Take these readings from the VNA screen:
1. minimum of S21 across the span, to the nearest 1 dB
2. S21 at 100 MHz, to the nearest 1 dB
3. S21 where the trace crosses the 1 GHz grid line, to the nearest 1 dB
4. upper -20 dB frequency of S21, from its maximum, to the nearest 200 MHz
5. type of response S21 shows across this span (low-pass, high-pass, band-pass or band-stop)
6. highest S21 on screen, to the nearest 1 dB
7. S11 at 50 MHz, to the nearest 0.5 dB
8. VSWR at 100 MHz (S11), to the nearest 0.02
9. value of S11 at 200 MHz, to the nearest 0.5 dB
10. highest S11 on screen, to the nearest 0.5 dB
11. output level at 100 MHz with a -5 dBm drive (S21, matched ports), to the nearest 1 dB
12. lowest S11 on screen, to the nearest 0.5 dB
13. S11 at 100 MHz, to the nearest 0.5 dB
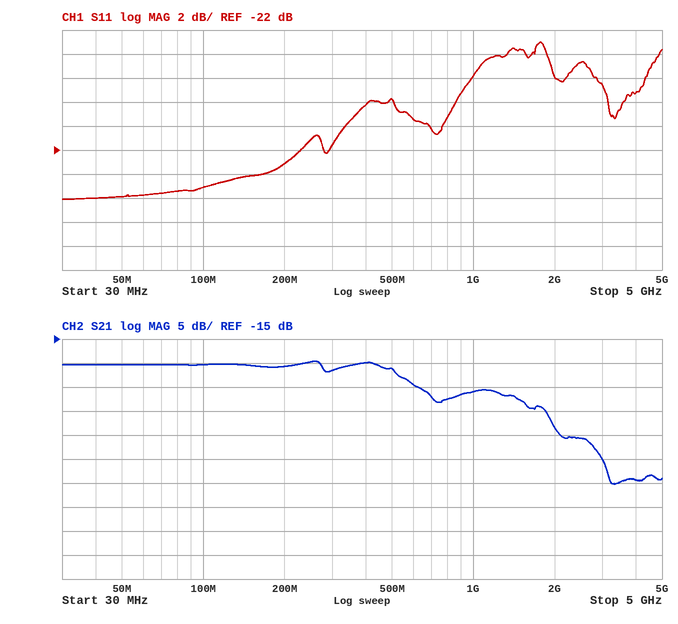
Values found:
-45 dB
-20 dB
-26 dB
3.0 GHz
low-pass
-20 dB
-26.0 dB
1.12
-23.0 dB
-13.0 dB
-25 dBm
-26.0 dB
-25.0 dB
